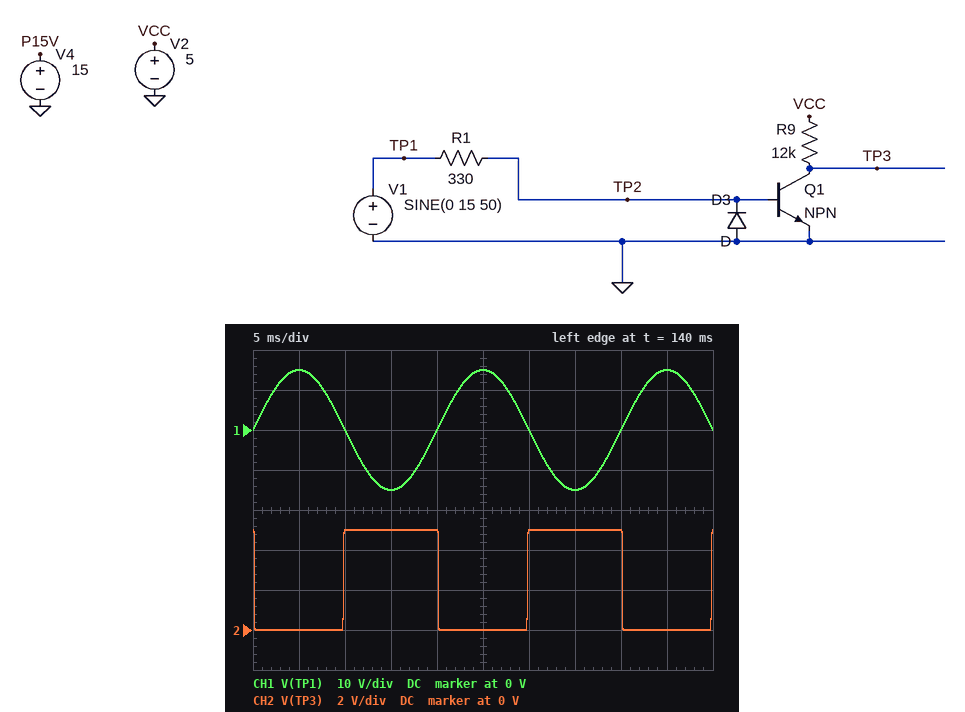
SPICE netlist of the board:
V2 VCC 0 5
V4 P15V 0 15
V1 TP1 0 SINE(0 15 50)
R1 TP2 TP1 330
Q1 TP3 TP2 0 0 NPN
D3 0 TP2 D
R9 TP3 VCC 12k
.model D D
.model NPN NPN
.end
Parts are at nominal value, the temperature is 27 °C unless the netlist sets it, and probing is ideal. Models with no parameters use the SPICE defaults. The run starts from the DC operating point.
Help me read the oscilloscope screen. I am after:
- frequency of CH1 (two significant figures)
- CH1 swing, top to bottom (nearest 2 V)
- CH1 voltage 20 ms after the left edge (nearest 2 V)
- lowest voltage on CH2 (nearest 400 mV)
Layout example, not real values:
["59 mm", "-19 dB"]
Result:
["50 Hz", "30 V", "0 V", "0 V"]
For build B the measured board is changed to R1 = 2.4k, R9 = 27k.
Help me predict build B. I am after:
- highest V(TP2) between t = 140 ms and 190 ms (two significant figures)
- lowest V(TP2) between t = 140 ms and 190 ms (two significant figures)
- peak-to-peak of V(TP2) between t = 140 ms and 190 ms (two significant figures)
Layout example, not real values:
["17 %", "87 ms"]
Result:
["840 mV", "-700 mV", "1.5 V"]
